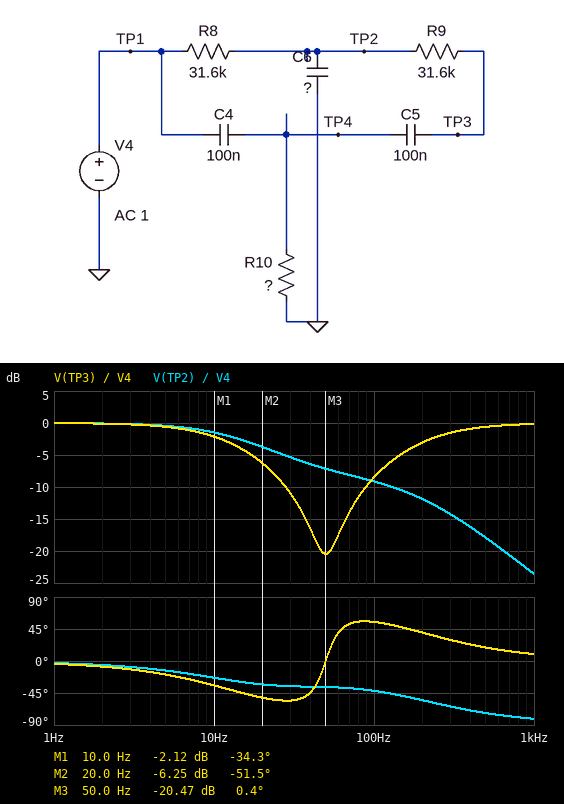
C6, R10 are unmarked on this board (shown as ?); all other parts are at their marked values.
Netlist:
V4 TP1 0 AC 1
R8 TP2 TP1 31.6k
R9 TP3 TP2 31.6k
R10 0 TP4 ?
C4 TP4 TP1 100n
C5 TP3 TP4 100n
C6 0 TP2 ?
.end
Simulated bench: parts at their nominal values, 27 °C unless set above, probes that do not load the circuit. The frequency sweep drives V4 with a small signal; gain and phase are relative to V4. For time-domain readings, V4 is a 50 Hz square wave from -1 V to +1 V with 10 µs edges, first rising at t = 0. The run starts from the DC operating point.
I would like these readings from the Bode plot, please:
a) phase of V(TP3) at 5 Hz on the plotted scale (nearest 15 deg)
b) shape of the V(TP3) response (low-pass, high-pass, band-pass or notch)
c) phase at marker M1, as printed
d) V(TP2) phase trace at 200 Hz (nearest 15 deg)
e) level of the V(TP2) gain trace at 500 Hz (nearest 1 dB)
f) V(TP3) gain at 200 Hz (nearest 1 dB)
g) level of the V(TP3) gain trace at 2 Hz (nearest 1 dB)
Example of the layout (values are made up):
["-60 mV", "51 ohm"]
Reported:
["-15 deg", "notch", "-34.3 deg", "-60 deg", "-18 dB", "-3 dB", "0 dB"]
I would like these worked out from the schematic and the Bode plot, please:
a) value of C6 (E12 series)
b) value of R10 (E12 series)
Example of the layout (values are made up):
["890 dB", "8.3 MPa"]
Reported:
["150 nF", "22 kΩ"]
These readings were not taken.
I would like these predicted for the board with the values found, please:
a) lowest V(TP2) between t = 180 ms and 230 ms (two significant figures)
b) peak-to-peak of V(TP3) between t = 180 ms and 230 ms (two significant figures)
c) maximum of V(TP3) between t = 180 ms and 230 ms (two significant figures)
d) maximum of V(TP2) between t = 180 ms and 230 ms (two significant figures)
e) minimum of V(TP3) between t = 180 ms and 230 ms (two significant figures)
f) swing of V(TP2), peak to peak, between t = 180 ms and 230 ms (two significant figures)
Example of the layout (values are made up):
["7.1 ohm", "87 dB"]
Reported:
["-610 mV", "3.2 V", "1.6 V", "610 mV", "-1.6 V", "1.2 V"]
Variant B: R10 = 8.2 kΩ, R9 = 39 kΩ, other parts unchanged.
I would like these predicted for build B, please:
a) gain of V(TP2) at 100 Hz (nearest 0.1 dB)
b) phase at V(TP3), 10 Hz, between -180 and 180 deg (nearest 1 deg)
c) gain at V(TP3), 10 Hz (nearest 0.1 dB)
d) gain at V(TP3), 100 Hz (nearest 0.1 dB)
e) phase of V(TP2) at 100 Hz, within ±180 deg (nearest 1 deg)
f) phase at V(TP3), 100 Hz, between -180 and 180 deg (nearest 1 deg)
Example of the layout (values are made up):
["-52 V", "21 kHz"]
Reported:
["-10.6 dB", "-38 deg", "-1.8 dB", "-12.4 dB", "-48 deg", "87 deg"]
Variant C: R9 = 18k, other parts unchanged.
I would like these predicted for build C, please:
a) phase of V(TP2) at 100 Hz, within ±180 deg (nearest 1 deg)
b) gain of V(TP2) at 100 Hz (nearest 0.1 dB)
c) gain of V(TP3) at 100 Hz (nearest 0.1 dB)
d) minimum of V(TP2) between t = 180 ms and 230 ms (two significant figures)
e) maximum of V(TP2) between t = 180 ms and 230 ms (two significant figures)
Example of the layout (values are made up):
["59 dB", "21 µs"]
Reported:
["-34 deg", "-9.6 dB", "-12.2 dB", "-580 mV", "580 mV"]
